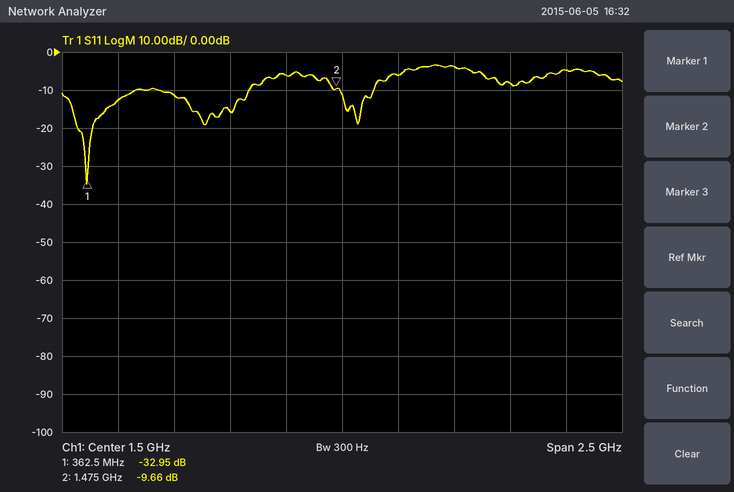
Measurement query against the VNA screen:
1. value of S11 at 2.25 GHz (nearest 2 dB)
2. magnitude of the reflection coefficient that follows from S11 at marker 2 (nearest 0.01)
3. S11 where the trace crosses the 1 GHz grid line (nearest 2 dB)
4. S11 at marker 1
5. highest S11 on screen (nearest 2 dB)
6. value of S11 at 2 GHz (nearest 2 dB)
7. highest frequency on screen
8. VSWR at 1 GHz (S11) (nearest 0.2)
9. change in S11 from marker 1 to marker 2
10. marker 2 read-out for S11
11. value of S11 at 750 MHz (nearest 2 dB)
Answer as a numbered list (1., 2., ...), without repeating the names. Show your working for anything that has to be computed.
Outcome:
1. -8 dB
2. 10^(-9.66/20) ≈ 0.33
3. -16 dB
4. -32.95 dB
5. -4 dB
6. -4 dB
7. 2.75 GHz
8. |Γ| = 10^(-16/20) = 0.1585; VSWR = (1 + 0.1585)/(1 − 0.1585) ≈ 1.4
9. -9.66 − (-32.95) = 23.29 dB
10. -9.66 dB
11. -12 dB
